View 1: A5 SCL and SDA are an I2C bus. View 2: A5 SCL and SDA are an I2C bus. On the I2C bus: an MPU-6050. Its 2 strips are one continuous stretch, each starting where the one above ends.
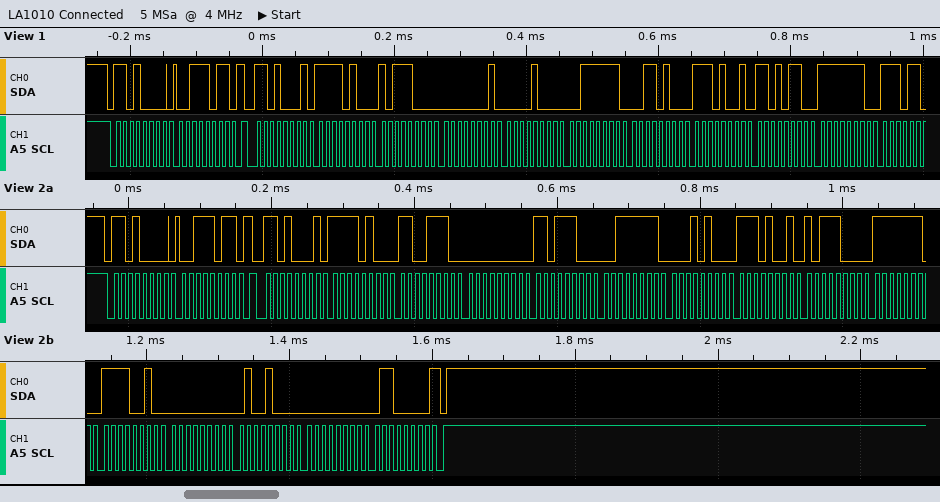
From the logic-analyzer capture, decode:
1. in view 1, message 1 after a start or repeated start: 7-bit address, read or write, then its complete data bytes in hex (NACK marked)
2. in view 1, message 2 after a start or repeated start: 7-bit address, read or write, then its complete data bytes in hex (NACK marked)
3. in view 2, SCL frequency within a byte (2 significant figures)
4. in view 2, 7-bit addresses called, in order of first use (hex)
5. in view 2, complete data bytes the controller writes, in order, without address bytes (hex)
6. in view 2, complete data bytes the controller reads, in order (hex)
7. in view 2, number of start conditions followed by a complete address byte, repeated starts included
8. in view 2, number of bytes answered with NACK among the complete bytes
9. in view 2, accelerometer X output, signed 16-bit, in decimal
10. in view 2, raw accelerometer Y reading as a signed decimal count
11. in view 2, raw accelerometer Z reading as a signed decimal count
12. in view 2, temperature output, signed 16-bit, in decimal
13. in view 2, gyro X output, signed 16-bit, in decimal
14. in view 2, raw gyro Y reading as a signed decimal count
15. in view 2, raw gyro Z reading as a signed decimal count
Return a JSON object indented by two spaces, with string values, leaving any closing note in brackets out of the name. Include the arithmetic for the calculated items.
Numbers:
{
  "in view 1, message 1 after a start or repeated start: 7-bit address, read or write, then its complete data bytes in hex": "0x68 write: 3B",
  "in view 1, message 2 after a start or repeated start: 7-bit address, read or write, then its complete data bytes in hex": "0x68 read: F4 B8 01 08 3F 34 E9 D6 FE",
  "in view 2, SCL frequency within a byte": "100 kHz",
  "in view 2, 7-bit addresses called, in order of first use": "0x68",
  "in view 2, complete data bytes the controller writes, in order, without address bytes": "3B",
  "in view 2, complete data bytes the controller reads, in order": "F4 CE 00 DC 3F 14 E9 B8 FE F2 00 48 00 60",
  "in view 2, number of start conditions followed by a complete address byte, repeated starts included": "2",
  "in view 2, number of bytes answered with NACK among the complete bytes": "1",
  "in view 2, accelerometer X output, signed 16-bit, in decimal": "0xF4CE = -2866",
  "in view 2, raw accelerometer Y reading as a signed decimal count": "0x00DC = 220",
  "in view 2, raw accelerometer Z reading as a signed decimal count": "0x3F14 = 16148",
  "in view 2, temperature output, signed 16-bit, in decimal": "0xE9B8 = -5704",
  "in view 2, gyro X output, signed 16-bit, in decimal": "0xFEF2 = -270",
  "in view 2, raw gyro Y reading as a signed decimal count": "0x0048 = 72",
  "in view 2, raw gyro Z reading as a signed decimal count": "0x0060 = 96"
}
